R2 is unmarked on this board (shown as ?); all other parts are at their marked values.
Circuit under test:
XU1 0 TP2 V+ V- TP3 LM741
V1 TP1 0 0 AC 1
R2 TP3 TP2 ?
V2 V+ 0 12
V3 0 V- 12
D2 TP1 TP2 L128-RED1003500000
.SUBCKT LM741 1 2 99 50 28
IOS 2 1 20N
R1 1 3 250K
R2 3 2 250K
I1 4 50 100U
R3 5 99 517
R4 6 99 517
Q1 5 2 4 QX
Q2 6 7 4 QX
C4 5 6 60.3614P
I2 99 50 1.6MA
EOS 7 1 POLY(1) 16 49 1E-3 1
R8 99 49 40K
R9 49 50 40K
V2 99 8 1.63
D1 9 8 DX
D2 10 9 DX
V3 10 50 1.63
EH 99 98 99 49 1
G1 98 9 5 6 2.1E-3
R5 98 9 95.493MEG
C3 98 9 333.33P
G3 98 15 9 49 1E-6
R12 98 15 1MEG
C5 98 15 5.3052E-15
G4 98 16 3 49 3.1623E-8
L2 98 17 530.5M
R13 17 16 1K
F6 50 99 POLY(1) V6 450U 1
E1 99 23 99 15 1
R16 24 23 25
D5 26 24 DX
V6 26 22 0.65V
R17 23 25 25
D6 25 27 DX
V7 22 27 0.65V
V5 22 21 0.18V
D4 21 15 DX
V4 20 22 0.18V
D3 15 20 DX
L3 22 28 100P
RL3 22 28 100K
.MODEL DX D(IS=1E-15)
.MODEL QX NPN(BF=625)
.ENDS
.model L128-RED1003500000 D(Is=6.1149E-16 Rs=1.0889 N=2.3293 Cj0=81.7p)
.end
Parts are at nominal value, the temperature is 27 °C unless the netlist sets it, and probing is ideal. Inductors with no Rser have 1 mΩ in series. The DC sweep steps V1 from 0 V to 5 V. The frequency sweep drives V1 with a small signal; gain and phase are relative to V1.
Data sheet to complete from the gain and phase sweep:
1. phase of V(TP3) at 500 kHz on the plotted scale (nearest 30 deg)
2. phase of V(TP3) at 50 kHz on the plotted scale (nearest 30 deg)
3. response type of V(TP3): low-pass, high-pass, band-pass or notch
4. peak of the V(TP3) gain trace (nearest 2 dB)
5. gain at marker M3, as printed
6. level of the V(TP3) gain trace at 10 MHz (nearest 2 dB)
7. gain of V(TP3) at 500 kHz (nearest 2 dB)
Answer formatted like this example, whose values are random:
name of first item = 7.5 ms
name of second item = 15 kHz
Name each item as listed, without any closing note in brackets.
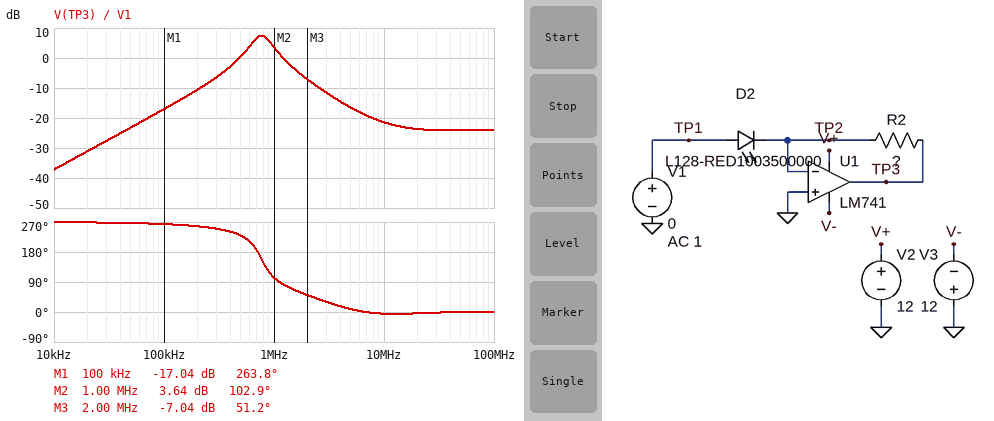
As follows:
phase of V(TP3) at 500 kHz on the plotted scale = 240 deg
phase of V(TP3) at 50 kHz on the plotted scale = 270 deg
response type of V(TP3): low-pass, high-pass, band-pass or notch = band-pass
peak of the V(TP3) gain trace = 8 dB
gain at marker M3, as printed = -7.04 dB
level of the V(TP3) gain trace at 10 MHz = -22 dB
gain of V(TP3) at 500 kHz = 0 dB
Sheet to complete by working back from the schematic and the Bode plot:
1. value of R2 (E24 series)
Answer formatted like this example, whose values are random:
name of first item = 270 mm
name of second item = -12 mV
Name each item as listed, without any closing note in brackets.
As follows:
value of R2 = 2.7 kΩ
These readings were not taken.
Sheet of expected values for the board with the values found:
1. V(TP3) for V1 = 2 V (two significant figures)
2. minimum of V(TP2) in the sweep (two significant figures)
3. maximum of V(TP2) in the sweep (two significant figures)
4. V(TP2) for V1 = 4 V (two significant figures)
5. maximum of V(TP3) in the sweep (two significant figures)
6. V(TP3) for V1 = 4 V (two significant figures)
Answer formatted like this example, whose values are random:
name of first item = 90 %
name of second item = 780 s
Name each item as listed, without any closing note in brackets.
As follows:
V(TP3) for V1 = 2 V = -11 V
minimum of V(TP2) in the sweep = 1.0 mV
maximum of V(TP2) in the sweep = 3.2 V
V(TP2) for V1 = 4 V = 2.2 V
maximum of V(TP3) in the sweep = 1.3 mV
V(TP3) for V1 = 4 V = -11 V
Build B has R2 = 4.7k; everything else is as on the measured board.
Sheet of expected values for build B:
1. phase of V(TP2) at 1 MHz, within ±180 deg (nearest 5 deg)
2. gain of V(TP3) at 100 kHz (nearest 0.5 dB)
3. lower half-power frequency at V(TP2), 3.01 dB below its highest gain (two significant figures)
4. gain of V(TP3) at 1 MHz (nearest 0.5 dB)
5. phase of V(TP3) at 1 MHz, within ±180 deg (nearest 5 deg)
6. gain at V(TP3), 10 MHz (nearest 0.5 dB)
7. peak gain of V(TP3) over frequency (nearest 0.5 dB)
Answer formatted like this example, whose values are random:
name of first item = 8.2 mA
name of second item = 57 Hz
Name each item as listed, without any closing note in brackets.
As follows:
phase of V(TP2) at 1 MHz, within ±180 deg = 20 deg
gain of V(TP3) at 100 kHz = -12.0 dB
lower half-power frequency at V(TP2), 3.01 dB below its highest gain = 540 kHz
gain of V(TP3) at 1 MHz = 2.0 dB
phase of V(TP3) at 1 MHz, within ±180 deg = 80 deg
gain at V(TP3), 10 MHz = -24.5 dB
peak gain of V(TP3) over frequency = 12.5 dB
